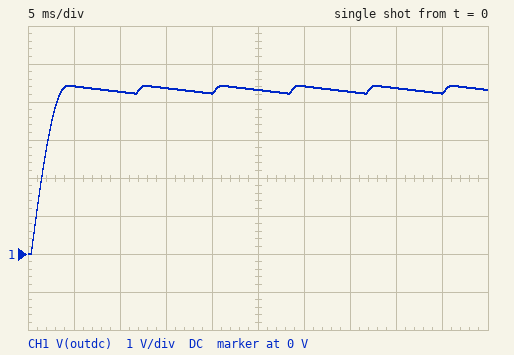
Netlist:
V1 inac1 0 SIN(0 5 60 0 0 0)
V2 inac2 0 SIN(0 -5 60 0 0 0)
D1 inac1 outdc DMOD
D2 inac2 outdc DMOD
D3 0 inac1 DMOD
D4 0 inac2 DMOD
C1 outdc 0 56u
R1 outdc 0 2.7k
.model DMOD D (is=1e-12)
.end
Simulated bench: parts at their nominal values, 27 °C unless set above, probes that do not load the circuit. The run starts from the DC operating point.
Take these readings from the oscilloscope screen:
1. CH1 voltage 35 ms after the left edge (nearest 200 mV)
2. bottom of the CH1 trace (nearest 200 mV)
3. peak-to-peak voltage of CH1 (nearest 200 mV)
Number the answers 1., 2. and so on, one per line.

1. 4.2 V
2. 0 V
3. 4.4 V
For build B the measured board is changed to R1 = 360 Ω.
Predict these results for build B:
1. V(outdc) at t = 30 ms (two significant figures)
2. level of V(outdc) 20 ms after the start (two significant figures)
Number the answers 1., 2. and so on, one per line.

1. 4.3 V
2. 4.1 V
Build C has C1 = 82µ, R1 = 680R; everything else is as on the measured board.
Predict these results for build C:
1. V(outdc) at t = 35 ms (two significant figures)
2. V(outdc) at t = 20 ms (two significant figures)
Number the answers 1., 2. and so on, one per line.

1. 4.0 V
2. 4.1 V
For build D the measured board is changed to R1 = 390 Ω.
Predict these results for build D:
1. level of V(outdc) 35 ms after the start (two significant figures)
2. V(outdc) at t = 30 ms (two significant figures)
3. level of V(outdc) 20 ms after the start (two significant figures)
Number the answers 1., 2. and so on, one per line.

1. 3.4 V
2. 4.3 V
3. 4.1 V
